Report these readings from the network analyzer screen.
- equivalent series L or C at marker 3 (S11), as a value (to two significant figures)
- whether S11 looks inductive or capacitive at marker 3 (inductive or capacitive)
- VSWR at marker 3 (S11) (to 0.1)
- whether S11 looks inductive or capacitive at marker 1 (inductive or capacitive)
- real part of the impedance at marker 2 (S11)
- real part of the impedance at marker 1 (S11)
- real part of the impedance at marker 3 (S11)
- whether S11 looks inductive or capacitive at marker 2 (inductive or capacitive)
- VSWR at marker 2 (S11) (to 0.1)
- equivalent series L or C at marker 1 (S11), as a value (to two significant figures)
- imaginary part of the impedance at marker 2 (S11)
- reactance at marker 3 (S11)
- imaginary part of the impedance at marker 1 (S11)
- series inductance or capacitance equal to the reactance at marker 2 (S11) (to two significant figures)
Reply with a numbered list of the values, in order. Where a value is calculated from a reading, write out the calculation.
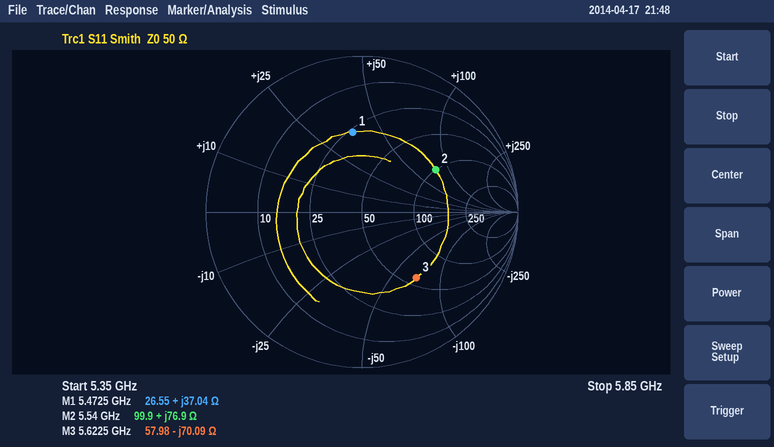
1. C = 1/(2π × 5.6225 GHz × 70.09 Ω) ≈ 404 fF, so 400 fF to two significant figures
2. capacitive
3. 3.4
4. inductive
5. 99.9 Ω
6. 26.55 Ω
7. 57.98 Ω
8. inductive
9. 3.4
10. L = 37.04 Ω/(2π × 5.4725 GHz) ≈ 1.1 nH
11. +76.9 Ω
12. -70.09 Ω
13. +37.04 Ω
14. L = 76.9 Ω/(2π × 5.54 GHz) ≈ 2.2 nH
